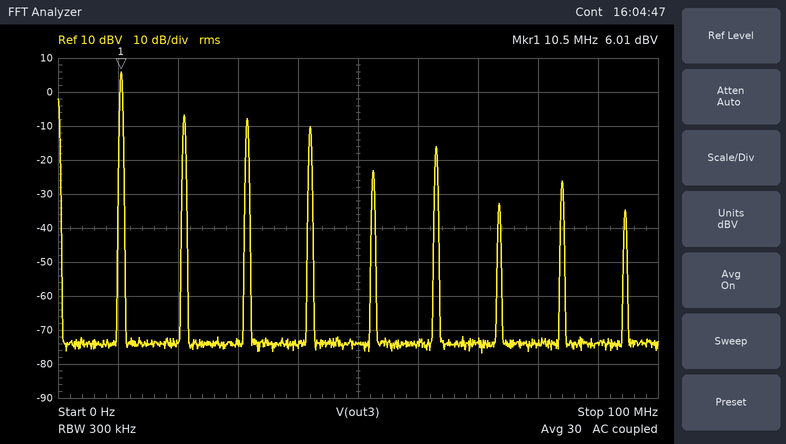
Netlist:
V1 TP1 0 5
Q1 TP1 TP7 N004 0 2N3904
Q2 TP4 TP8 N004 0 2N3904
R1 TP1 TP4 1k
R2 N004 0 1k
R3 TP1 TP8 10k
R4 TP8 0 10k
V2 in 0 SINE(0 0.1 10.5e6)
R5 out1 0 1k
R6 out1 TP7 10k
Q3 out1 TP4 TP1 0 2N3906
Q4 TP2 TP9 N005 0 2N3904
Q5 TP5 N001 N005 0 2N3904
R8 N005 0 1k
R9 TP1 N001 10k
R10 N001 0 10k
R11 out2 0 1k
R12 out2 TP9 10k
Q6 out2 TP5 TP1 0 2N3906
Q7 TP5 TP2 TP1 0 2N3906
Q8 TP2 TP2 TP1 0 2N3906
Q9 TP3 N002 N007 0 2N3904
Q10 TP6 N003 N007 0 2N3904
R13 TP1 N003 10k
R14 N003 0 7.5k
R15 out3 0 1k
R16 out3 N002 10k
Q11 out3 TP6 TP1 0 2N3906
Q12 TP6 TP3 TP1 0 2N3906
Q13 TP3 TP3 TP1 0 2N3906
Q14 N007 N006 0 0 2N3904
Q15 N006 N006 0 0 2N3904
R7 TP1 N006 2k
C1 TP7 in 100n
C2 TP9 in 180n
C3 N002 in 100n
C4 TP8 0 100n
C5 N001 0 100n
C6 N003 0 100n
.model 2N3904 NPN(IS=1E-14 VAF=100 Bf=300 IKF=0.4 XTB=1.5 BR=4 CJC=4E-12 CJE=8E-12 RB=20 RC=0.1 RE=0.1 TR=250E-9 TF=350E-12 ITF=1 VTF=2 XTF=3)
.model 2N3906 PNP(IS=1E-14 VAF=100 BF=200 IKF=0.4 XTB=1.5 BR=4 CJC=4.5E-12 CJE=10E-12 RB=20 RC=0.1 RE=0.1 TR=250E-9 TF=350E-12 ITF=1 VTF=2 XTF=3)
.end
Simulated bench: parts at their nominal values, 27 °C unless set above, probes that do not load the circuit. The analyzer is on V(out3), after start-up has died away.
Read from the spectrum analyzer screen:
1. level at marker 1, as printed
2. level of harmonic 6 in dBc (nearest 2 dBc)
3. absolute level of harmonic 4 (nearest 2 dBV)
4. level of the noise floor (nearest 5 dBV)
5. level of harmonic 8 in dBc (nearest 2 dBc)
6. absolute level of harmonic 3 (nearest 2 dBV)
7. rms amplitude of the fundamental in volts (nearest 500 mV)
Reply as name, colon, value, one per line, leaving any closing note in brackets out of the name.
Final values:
level at marker 1, as printed: 6.01 dBV
level of harmonic 6 in dBc: -22 dBc
absolute level of harmonic 4: -10 dBV
level of the noise floor: -75 dBV
level of harmonic 8 in dBc: -32 dBc
absolute level of harmonic 3: -8 dBV
rms amplitude of the fundamental in volts: 2.0 V
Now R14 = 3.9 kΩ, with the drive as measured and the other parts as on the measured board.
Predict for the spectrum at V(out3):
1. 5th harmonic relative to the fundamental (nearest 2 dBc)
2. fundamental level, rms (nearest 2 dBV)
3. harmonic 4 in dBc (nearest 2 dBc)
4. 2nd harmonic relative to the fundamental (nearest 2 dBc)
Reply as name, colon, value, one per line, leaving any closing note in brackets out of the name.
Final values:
5th harmonic relative to the fundamental: -18 dBc
fundamental level, rms: 4 dBV
harmonic 4 in dBc: -24 dBc
2nd harmonic relative to the fundamental: -4 dBc
